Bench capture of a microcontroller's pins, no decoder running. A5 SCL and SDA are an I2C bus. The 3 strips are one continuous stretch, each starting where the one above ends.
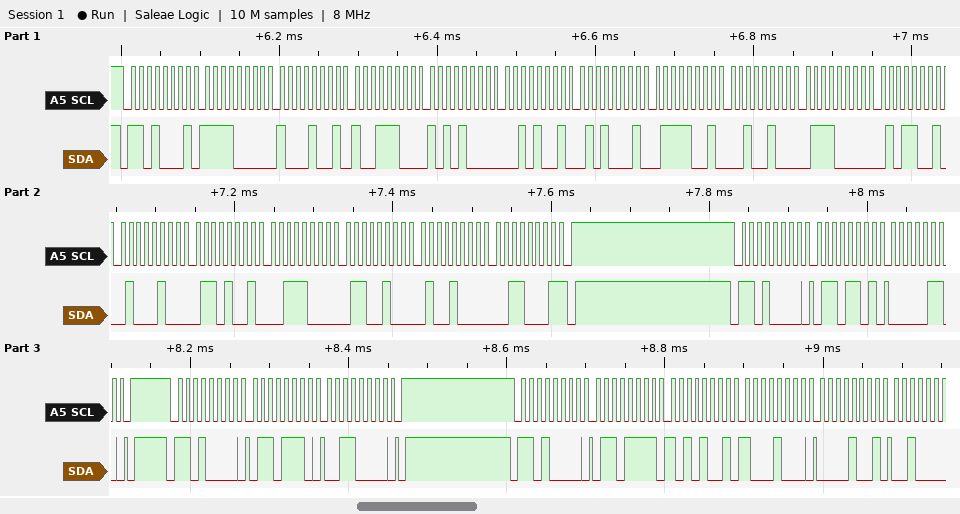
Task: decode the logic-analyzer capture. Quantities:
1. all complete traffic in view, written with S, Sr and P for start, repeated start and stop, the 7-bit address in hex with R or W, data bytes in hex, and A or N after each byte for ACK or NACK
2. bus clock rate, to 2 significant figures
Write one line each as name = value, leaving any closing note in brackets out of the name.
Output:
all complete traffic in view, written with S, Sr and P for start, repeated start and stop, the 7-bit address in hex with R or W, data bytes in hex, and A or N after each byte for ACK or NACK = S 68R A F0 A 89 A 9C A A8 A 29 A 51 A 79 A 24 A 70 A 59 A 44 A 69 A 38 A 64 A 48 A 31 N P S 68W A 6D A 06 A P S 68W A 6E A 30 A P S 68W A 6F A A9 A 88 A 09 A
bus clock rate, to 2 significant figures = 100 kHz
